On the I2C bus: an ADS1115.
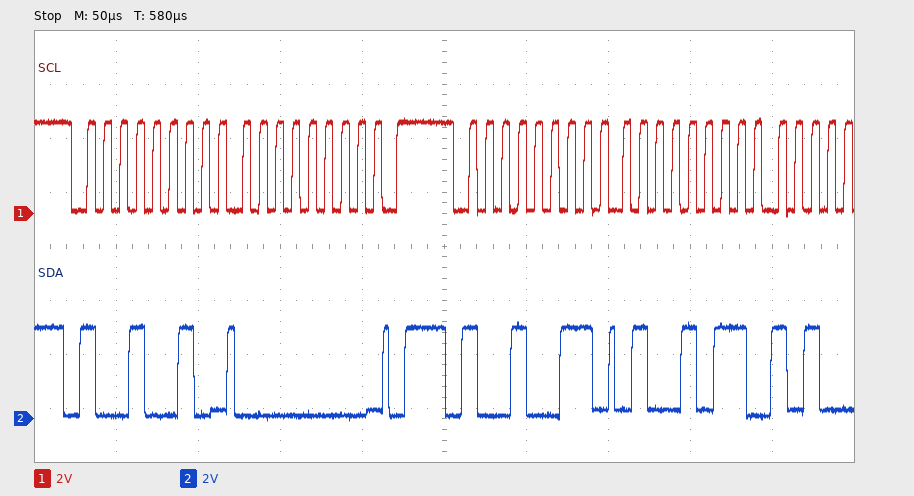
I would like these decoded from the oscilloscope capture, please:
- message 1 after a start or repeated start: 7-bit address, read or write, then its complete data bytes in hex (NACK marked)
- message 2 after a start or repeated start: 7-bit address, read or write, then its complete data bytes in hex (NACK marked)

0x49 write: 00
0x49 read: 4B
